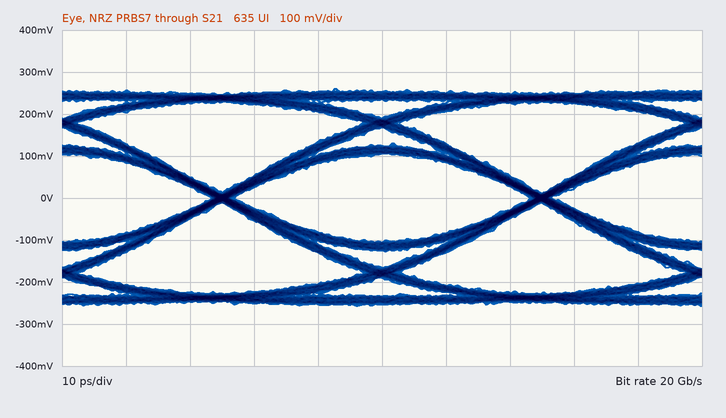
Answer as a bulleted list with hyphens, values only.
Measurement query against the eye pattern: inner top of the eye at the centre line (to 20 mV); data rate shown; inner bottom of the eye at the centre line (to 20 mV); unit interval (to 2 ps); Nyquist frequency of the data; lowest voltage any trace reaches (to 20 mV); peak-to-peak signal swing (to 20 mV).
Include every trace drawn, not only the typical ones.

- 100 mV
- 20 Gb/s
- -100 mV
- 50 ps
- 10 GHz
- -260 mV
- 520 mV
